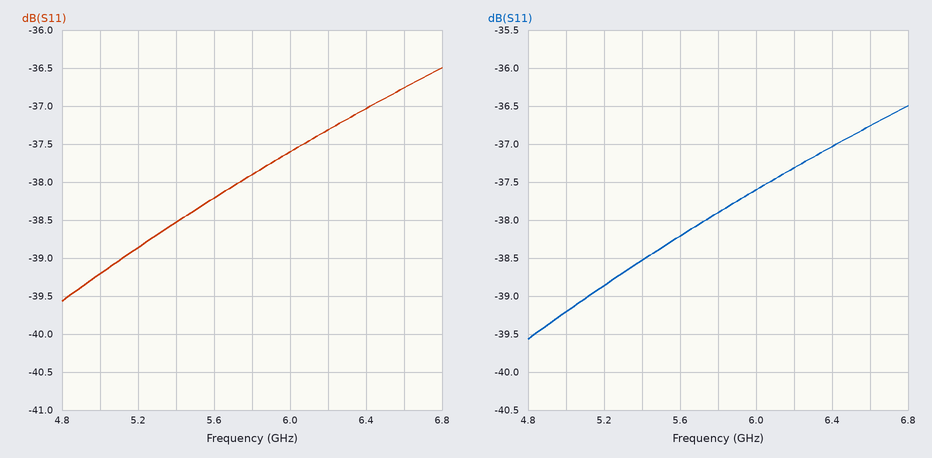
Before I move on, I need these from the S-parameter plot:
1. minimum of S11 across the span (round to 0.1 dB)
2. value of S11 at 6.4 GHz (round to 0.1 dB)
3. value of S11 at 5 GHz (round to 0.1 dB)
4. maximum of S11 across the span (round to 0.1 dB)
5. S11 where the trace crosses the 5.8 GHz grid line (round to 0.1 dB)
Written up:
-39.6 dB
-37.0 dB
-39.2 dB
-36.5 dB
-37.9 dB
